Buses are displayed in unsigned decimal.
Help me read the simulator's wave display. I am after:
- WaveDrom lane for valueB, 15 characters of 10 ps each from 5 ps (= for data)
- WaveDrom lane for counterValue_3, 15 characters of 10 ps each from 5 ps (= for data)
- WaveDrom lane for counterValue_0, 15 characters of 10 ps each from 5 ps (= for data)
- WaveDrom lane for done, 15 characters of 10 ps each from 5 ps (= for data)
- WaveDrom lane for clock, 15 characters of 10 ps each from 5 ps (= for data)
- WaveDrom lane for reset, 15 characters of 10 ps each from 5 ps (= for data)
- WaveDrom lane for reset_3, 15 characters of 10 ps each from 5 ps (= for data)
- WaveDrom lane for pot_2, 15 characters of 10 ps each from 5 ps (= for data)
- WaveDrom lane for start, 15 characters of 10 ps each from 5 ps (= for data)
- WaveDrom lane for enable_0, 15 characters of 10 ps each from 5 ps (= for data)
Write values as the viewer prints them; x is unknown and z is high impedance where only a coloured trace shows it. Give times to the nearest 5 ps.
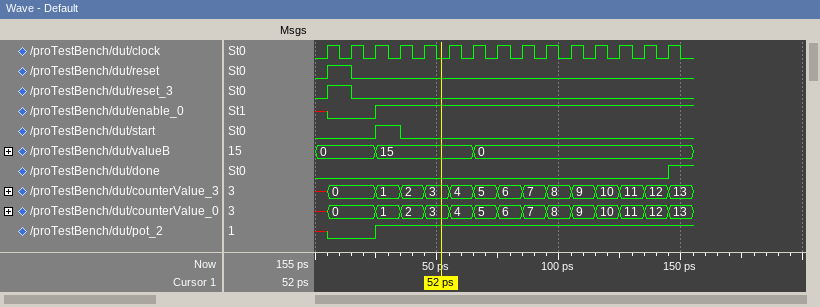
{name: 'valueB', wave: '=.=...=........', data: '0 15 0'}
{name: 'counterValue_3', wave: '=.=============', data: '0 1 2 3 4 5 6 7 8 9 10 11 12 13'}
{name: 'counterValue_0', wave: '=.=============', data: '0 1 2 3 4 5 6 7 8 9 10 11 12 13'}
{name: 'done', wave: '0.............1'}
{name: 'clock', wave: 'p..............'}
{name: 'reset', wave: '10.............'}
{name: 'reset_3', wave: '10.............'}
{name: 'pot_2', wave: '0.1............'}
{name: 'start', wave: '0.10...........'}
{name: 'enable_0', wave: '0.1............'}
